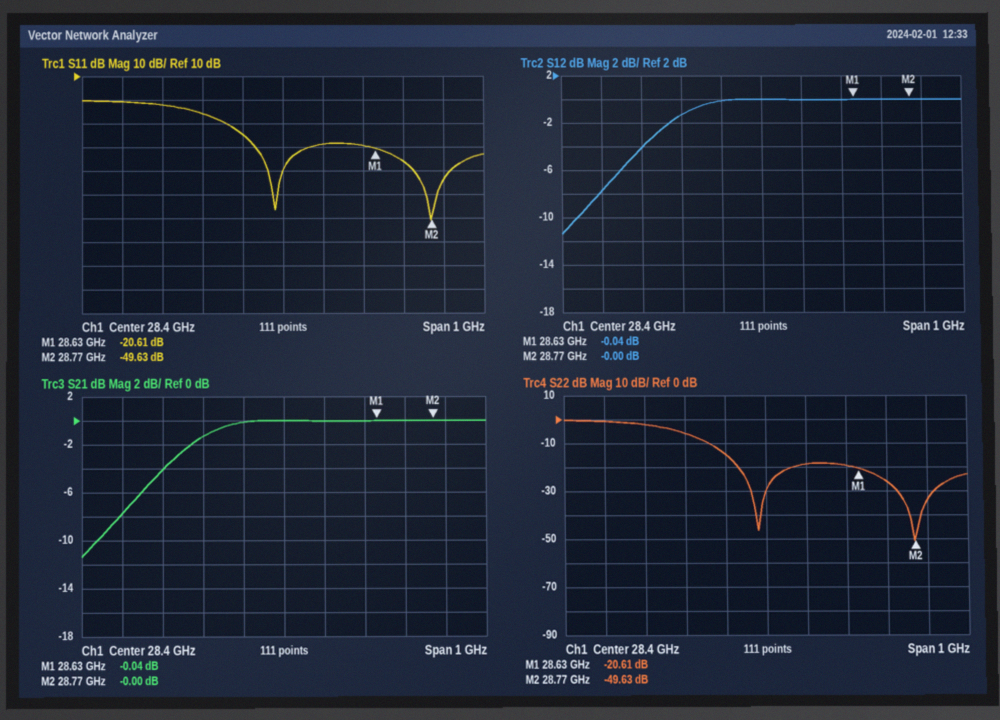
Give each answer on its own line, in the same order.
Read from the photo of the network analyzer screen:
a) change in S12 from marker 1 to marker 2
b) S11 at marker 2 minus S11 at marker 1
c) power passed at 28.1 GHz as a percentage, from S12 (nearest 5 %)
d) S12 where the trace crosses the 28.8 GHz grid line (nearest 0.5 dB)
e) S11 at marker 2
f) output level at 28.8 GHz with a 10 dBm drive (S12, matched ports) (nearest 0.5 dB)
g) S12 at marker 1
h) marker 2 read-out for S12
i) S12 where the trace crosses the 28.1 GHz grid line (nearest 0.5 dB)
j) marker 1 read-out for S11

0.04 dB
-29.02 dB
40 %
0.0 dB
-49.63 dB
10.0 dBm
-0.04 dB
-0.00 dB
-4.0 dB
-20.61 dB
